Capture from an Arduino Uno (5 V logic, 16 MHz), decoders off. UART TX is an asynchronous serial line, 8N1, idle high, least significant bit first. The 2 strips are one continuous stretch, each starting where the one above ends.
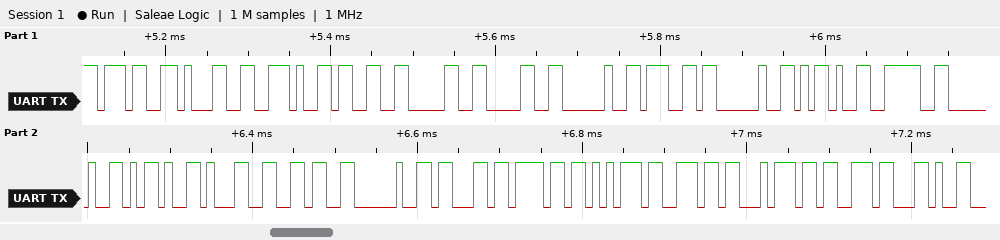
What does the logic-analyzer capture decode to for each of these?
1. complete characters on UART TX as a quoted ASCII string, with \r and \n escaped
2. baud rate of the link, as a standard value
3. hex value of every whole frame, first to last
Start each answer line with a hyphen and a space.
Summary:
- "71.300 g -> -16 counts,"
- 115200 baud
- 37 31 2E 33 30 30 20 67 20 2D 3E 20 2D 31 36 20 63 6F 75 6E 74 73 2C
